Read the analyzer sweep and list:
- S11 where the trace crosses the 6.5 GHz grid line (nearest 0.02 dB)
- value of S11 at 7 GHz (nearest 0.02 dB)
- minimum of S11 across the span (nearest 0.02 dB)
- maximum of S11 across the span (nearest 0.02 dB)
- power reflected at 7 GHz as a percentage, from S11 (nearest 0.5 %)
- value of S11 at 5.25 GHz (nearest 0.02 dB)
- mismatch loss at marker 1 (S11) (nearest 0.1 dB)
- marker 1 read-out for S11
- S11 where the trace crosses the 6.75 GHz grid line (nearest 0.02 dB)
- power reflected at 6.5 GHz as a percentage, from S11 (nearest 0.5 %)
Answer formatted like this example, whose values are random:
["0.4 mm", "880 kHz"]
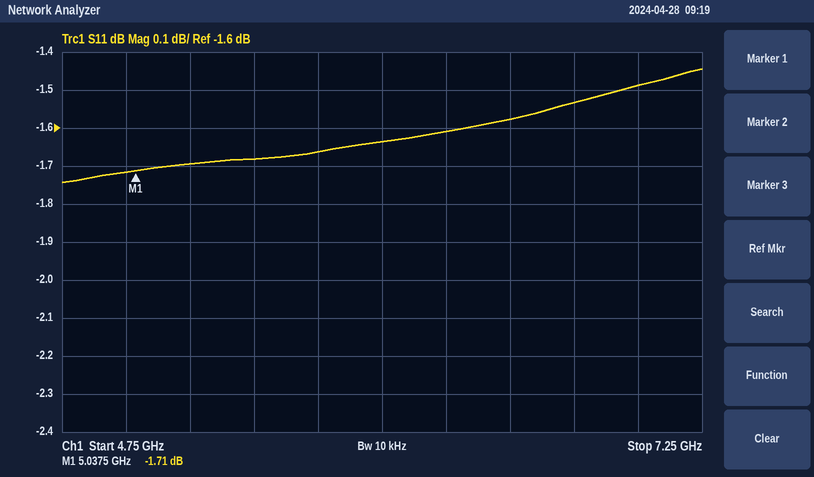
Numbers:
["-1.58 dB", "-1.48 dB", "-1.74 dB", "-1.44 dB", "71.0 %", "-1.70 dB", "4.9 dB", "-1.71 dB", "-1.54 dB", "69.5 %"]
